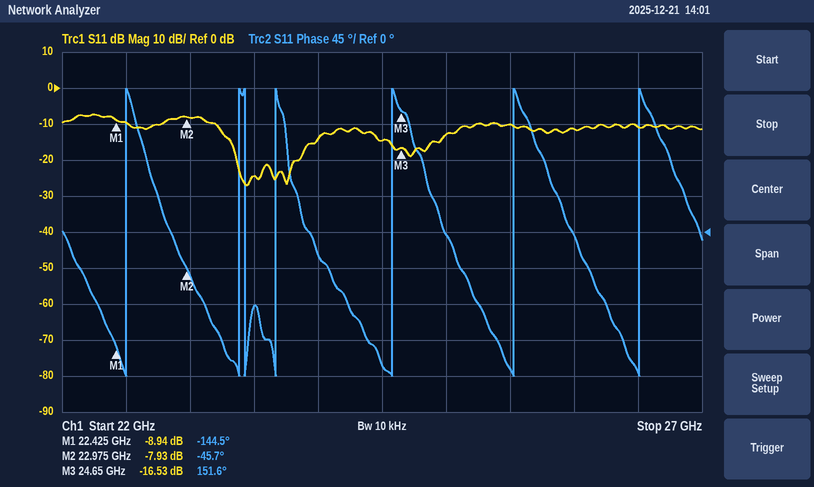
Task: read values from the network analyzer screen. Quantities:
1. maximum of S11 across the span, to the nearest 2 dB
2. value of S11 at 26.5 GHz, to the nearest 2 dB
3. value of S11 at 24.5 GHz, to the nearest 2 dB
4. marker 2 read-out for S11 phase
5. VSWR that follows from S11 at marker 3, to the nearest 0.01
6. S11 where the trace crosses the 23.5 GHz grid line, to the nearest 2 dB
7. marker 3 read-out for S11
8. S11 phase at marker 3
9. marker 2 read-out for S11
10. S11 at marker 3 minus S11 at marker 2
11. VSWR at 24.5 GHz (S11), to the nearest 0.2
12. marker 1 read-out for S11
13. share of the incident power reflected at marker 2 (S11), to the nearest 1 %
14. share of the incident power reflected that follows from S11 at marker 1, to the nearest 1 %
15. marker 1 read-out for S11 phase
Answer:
-8 dB
-10 dB
-14 dB
-45.7°
1.35
-24 dB
-16.53 dB
151.6°
-7.93 dB
-8.60 dB
1.4
-8.94 dB
16 %
13 %
-144.5°
